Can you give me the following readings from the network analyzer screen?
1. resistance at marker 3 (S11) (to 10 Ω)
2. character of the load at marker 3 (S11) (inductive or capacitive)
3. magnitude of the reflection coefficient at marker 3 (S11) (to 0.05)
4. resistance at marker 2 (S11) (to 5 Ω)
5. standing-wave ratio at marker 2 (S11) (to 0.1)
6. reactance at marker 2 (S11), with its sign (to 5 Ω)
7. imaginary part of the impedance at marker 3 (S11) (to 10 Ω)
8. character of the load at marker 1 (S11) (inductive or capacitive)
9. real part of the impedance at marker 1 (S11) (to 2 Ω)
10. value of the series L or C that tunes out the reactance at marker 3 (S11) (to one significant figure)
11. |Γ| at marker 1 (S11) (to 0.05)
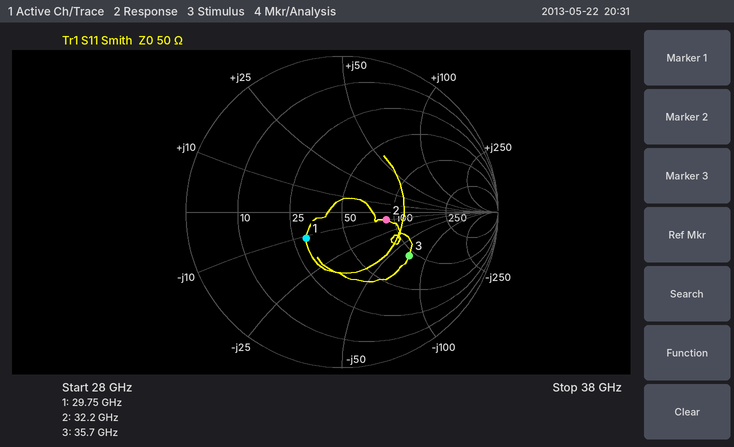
90 Ω
capacitive
0.50
90 Ω
1.8
-10 Ω
-70 Ω
capacitive
30 Ω
300 pH
0.30
